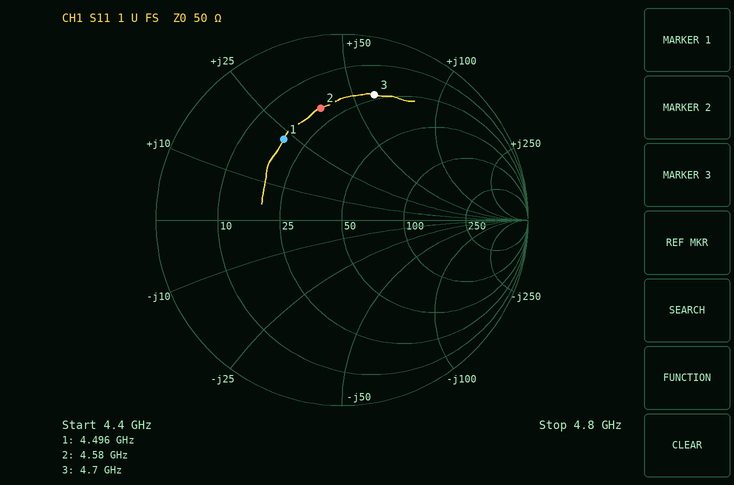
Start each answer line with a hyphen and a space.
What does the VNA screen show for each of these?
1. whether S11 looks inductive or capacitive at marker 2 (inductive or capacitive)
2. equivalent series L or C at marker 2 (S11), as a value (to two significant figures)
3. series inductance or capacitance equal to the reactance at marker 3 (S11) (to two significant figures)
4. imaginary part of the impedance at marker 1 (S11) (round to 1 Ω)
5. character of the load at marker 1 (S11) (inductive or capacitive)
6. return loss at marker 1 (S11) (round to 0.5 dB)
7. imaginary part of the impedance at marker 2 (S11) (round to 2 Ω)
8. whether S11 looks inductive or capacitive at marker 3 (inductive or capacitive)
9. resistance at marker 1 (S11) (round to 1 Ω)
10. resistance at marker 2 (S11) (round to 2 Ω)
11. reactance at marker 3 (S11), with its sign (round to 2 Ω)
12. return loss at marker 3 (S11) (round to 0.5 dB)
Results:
- inductive
- 1.3 nH
- 2.0 nH
- +23 Ω
- inductive
- 5.5 dB
- +38 Ω
- inductive
- 19 Ω
- 20 Ω
- +60 Ω
- 3.0 dB
